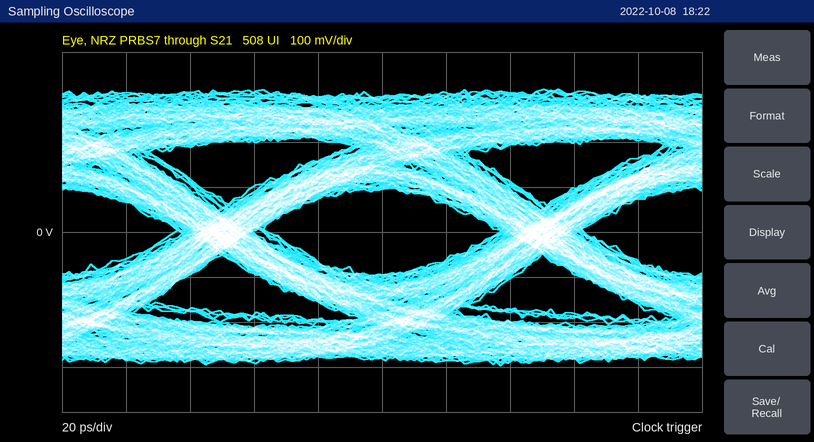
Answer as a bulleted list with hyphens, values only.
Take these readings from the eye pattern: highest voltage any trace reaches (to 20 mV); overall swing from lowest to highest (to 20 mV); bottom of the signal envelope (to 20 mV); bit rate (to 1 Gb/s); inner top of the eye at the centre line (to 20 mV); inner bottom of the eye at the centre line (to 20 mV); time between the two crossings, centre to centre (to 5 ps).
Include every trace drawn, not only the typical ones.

- 320 mV
- 620 mV
- -300 mV
- 10 Gb/s
- 100 mV
- -100 mV
- 100 ps
